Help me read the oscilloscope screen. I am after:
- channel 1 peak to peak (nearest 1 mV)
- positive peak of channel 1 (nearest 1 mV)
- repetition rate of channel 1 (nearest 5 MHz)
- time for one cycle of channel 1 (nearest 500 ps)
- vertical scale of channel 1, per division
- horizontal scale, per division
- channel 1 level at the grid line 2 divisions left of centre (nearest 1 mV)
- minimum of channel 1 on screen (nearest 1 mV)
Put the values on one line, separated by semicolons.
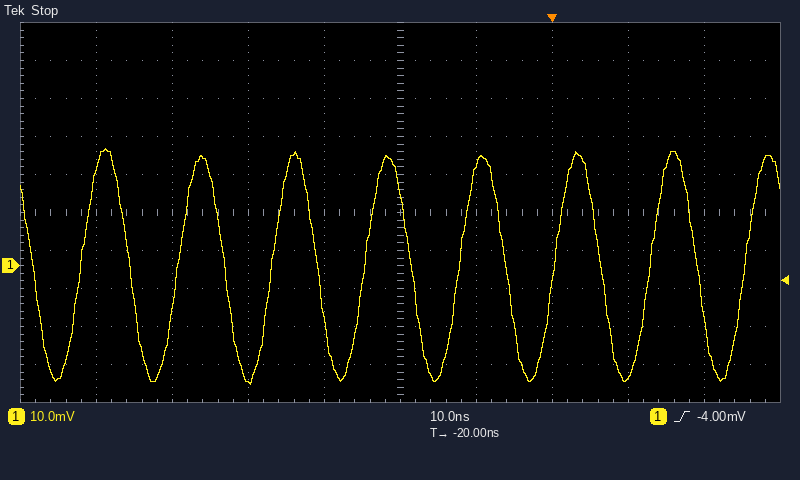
62 mV; 31 mV; 80 MHz; 12.5 ns; 10 mV; 10 ns; -30 mV; -31 mV
